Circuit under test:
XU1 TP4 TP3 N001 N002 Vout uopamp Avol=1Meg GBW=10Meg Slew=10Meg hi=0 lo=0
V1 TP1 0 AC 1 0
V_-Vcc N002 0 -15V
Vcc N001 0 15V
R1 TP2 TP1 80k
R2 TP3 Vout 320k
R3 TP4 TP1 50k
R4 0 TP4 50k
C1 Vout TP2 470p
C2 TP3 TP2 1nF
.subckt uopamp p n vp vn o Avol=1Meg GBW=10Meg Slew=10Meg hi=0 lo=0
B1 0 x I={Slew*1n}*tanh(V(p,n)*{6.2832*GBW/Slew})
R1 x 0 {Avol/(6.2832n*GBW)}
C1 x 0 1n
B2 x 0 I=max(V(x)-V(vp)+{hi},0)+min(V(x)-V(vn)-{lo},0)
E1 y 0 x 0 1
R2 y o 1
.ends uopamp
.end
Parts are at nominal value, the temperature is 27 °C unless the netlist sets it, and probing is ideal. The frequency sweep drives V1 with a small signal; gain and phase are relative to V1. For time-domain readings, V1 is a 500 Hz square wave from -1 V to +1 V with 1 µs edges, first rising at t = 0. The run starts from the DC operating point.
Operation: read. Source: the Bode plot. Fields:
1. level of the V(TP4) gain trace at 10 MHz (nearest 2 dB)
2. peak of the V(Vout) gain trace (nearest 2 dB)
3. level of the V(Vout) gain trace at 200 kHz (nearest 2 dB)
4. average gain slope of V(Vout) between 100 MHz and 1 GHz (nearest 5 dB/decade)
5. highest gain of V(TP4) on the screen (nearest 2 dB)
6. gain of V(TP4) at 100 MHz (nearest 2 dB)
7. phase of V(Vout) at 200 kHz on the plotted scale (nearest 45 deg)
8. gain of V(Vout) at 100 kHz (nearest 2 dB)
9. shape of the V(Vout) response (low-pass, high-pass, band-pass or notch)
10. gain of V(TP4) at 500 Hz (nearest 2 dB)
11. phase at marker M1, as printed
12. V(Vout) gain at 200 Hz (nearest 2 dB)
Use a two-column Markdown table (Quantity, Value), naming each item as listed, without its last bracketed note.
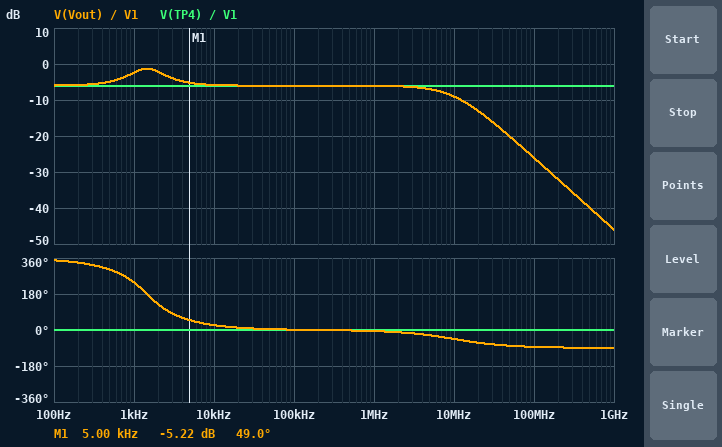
| Quantity | Value |
|---|---|
| level of the V(TP4) gain trace at 10 MHz | -6 dB |
| peak of the V(Vout) gain trace | -2 dB |
| level of the V(Vout) gain trace at 200 kHz | -6 dB |
| average gain slope of V(Vout) between 100 MHz and 1 GHz | -20 dB/decade |
| highest gain of V(TP4) on the screen | -6 dB |
| gain of V(TP4) at 100 MHz | -6 dB |
| phase of V(Vout) at 200 kHz on the plotted scale | 0 deg |
| gain of V(Vout) at 100 kHz | -6 dB |
| shape of the V(Vout) response | low-pass |
| gain of V(TP4) at 500 Hz | -6 dB |
| phase at marker M1, as printed | 49.0 deg |
| V(Vout) gain at 200 Hz | -6 dB |
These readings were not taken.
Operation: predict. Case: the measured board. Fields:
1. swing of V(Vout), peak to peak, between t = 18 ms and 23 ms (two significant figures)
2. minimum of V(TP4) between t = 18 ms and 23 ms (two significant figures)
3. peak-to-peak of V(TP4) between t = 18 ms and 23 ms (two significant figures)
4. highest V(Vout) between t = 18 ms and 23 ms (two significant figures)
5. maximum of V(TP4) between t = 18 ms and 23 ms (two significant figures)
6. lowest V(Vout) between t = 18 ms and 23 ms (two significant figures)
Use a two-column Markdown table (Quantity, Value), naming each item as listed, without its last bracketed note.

| Quantity | Value |
|---|---|
| swing of V(Vout), peak to peak, between t = 18 ms and 23 ms | 2.1 V |
| minimum of V(TP4) between t = 18 ms and 23 ms | -500 mV |
| peak-to-peak of V(TP4) between t = 18 ms and 23 ms | 1.0 V |
| highest V(Vout) between t = 18 ms and 23 ms | 1.0 V |
| maximum of V(TP4) between t = 18 ms and 23 ms | 500 mV |
| lowest V(Vout) between t = 18 ms and 23 ms | -1.0 V |
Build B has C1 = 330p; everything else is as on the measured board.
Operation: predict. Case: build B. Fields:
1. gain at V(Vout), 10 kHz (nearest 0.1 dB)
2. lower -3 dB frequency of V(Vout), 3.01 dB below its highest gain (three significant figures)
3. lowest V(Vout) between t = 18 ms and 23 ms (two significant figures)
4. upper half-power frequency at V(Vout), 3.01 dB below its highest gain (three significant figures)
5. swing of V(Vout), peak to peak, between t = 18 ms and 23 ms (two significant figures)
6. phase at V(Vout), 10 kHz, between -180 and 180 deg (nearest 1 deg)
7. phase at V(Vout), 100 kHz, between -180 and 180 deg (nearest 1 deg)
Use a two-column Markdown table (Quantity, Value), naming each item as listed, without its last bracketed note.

| Quantity | Value |
|---|---|
| gain at V(Vout), 10 kHz | -5.5 dB |
| lower -3 dB frequency of V(Vout), 3.01 dB below its highest gain | 822 Hz |
| lowest V(Vout) between t = 18 ms and 23 ms | -1.3 V |
| upper half-power frequency at V(Vout), 3.01 dB below its highest gain | 3.64 kHz |
| swing of V(Vout), peak to peak, between t = 18 ms and 23 ms | 2.5 V |
| phase at V(Vout), 10 kHz, between -180 and 180 deg | 34 deg |
| phase at V(Vout), 100 kHz, between -180 and 180 deg | 3 deg |
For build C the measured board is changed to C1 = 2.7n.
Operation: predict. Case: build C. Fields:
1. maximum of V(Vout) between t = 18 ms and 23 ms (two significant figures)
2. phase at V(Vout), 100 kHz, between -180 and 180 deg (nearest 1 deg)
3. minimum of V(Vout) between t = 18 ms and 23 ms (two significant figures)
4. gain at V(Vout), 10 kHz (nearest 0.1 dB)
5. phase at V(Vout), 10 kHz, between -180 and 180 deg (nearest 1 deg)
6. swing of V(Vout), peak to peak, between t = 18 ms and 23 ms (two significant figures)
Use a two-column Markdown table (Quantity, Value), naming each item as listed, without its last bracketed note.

| Quantity | Value |
|---|---|
| maximum of V(Vout) between t = 18 ms and 23 ms | 500 mV |
| phase at V(Vout), 100 kHz, between -180 and 180 deg | 0 deg |
| minimum of V(Vout) between t = 18 ms and 23 ms | -500 mV |
| gain at V(Vout), 10 kHz | -6.0 dB |
| phase at V(Vout), 10 kHz, between -180 and 180 deg | 4 deg |
| swing of V(Vout), peak to peak, between t = 18 ms and 23 ms | 1.0 V |
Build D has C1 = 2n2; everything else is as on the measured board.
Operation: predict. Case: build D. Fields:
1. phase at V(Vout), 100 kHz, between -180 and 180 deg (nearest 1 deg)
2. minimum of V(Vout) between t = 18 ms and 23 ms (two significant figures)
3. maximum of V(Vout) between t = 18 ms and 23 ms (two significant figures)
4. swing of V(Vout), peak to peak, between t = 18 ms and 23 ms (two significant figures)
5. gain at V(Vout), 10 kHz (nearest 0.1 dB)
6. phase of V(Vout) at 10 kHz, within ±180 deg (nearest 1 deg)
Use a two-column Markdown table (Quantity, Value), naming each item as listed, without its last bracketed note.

| Quantity | Value |
|---|---|
| phase at V(Vout), 100 kHz, between -180 and 180 deg | 0 deg |
| minimum of V(Vout) between t = 18 ms and 23 ms | -580 mV |
| maximum of V(Vout) between t = 18 ms and 23 ms | 580 mV |
| swing of V(Vout), peak to peak, between t = 18 ms and 23 ms | 1.2 V |
| gain at V(Vout), 10 kHz | -6.0 dB |
| phase of V(Vout) at 10 kHz, within ±180 deg | 5 deg |
